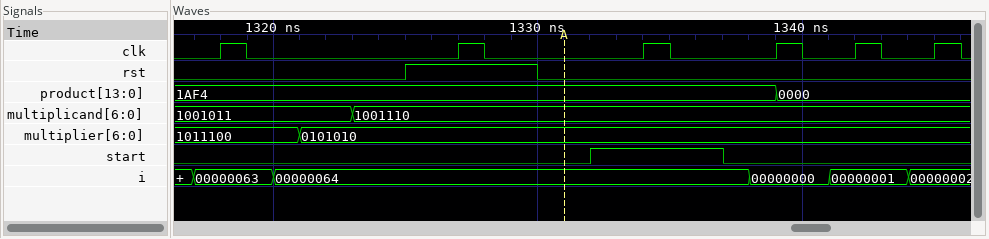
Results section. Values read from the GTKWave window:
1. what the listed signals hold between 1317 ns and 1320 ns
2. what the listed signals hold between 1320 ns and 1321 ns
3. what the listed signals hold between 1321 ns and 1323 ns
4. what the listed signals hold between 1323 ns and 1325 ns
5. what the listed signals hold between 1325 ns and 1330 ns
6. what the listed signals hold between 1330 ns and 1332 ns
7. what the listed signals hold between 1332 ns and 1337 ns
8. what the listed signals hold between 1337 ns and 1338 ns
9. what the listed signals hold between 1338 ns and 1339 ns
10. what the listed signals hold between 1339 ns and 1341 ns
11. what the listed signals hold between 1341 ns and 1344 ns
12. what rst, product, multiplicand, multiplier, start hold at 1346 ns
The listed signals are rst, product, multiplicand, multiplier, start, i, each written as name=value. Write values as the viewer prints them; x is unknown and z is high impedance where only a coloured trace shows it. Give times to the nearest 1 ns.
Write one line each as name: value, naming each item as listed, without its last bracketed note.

what the listed signals hold between 1317 ns and 1320 ns: rst=0, product=1AF4, multiplicand=1001011, multiplier=1011100, start=0, i=00000063
what the listed signals hold between 1320 ns and 1321 ns: rst=0, product=1AF4, multiplicand=1001011, multiplier=1011100, start=0, i=00000064
what the listed signals hold between 1321 ns and 1323 ns: rst=0, product=1AF4, multiplicand=1001011, multiplier=0101010, start=0, i=00000064
what the listed signals hold between 1323 ns and 1325 ns: rst=0, product=1AF4, multiplicand=1001110, multiplier=0101010, start=0, i=00000064
what the listed signals hold between 1325 ns and 1330 ns: rst=1, product=1AF4, multiplicand=1001110, multiplier=0101010, start=0, i=00000064
what the listed signals hold between 1330 ns and 1332 ns: rst=0, product=1AF4, multiplicand=1001110, multiplier=0101010, start=0, i=00000064
what the listed signals hold between 1332 ns and 1337 ns: rst=0, product=1AF4, multiplicand=1001110, multiplier=0101010, start=1, i=00000064
what the listed signals hold between 1337 ns and 1338 ns: rst=0, product=1AF4, multiplicand=1001110, multiplier=0101010, start=0, i=00000064
what the listed signals hold between 1338 ns and 1339 ns: rst=0, product=1AF4, multiplicand=1001110, multiplier=0101010, start=0, i=00000000
what the listed signals hold between 1339 ns and 1341 ns: rst=0, product=0000, multiplicand=1001110, multiplier=0101010, start=0, i=00000000
what the listed signals hold between 1341 ns and 1344 ns: rst=0, product=0000, multiplicand=1001110, multiplier=0101010, start=0, i=00000001
what rst, product, multiplicand, multiplier, start hold at 1346 ns: rst=0, product=0000, multiplicand=1001110, multiplier=0101010, start=0
